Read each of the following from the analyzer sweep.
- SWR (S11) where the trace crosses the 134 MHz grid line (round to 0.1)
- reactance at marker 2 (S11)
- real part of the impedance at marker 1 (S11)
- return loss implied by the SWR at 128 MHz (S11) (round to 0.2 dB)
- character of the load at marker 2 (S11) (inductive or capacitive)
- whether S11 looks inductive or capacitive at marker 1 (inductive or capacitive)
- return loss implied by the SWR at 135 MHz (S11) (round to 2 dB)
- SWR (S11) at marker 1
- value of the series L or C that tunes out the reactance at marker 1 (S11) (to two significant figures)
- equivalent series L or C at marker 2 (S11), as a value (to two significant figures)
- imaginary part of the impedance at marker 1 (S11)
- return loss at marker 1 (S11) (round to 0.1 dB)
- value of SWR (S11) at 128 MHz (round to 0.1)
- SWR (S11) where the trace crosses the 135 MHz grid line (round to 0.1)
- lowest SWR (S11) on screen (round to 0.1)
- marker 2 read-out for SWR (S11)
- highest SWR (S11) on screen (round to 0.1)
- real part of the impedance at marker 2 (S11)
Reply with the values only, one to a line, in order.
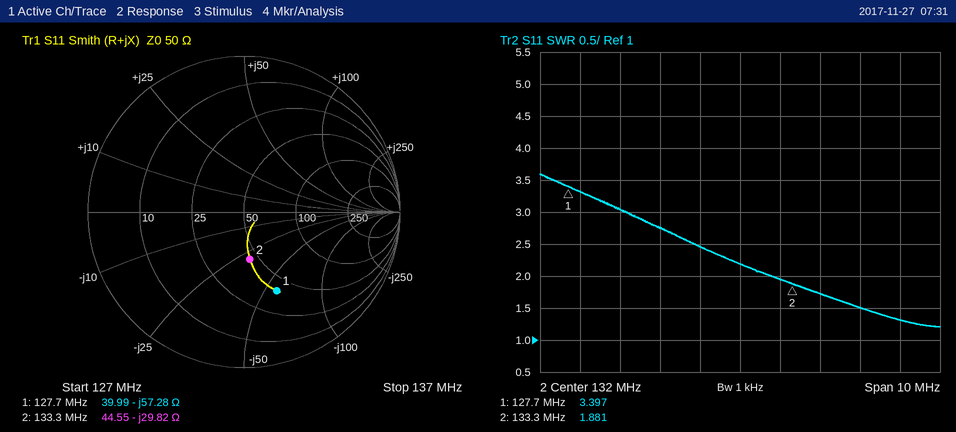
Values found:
1.7
-29.82 Ω
39.99 Ω
5.4 dB
capacitive
capacitive
14 dB
3.397
71 nH
40 pF
-57.28 Ω
5.3 dB
3.3
1.5
1.2
1.881
3.6
44.55 Ω
